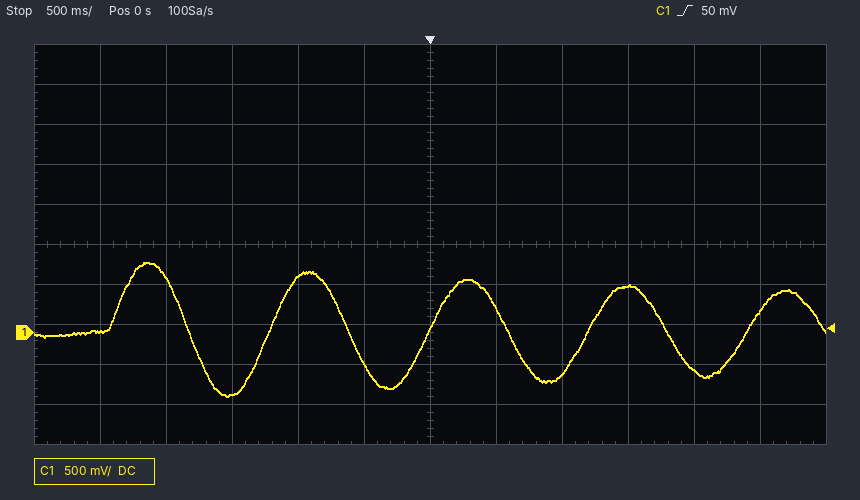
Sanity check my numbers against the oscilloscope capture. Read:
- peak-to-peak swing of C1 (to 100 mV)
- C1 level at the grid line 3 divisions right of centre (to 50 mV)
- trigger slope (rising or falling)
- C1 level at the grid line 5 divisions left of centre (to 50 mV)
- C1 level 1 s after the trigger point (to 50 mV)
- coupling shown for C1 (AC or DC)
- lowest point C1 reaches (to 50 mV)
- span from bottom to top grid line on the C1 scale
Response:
1.70 V
600 mV
rising
0 mV
-500 mV
DC
-800 mV
5 V
